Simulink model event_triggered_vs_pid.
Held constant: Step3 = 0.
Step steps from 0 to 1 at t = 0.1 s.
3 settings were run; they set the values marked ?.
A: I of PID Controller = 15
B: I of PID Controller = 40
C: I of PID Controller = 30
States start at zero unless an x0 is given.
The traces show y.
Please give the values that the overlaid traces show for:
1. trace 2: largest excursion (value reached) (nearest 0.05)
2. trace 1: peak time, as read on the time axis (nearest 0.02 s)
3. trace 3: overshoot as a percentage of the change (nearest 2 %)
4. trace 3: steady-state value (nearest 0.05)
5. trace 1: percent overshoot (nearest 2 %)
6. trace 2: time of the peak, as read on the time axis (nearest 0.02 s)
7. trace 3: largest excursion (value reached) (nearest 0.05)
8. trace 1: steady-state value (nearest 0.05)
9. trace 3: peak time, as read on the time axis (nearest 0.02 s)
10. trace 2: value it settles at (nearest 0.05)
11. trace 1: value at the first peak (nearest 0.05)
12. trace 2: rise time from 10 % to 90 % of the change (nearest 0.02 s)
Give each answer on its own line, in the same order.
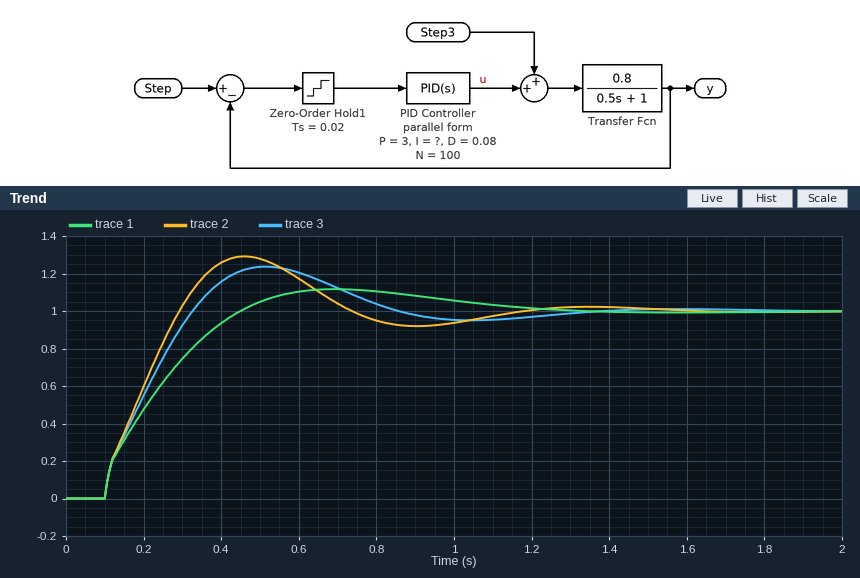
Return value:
1.30
0.70 s
24 %
1.00
12 %
0.46 s
1.25
1.00
0.52 s
1.00
1.10
0.16 s
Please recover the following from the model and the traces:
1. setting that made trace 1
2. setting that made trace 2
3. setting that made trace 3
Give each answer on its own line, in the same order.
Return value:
A
B
C
